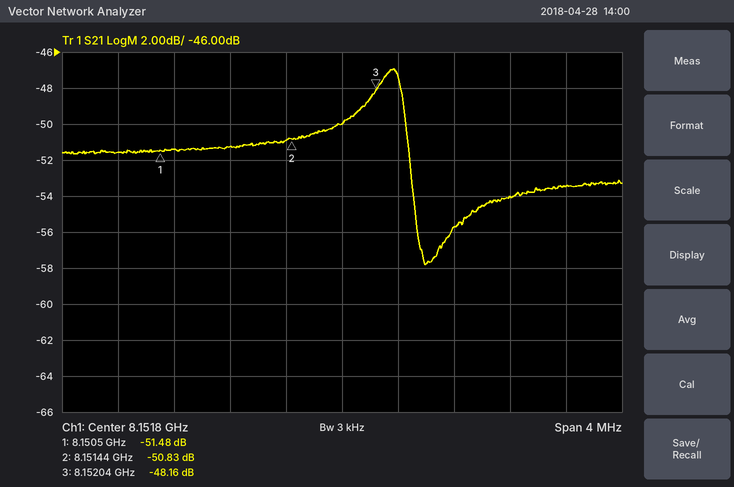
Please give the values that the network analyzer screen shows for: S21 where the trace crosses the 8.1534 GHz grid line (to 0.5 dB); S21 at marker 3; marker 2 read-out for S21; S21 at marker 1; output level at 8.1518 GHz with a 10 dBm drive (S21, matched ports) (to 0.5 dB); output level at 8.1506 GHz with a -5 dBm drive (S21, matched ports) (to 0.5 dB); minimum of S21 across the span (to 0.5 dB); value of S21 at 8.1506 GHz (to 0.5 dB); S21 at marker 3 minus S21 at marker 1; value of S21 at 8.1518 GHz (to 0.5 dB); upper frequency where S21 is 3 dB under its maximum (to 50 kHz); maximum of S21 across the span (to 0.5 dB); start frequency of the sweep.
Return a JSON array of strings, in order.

["-53.5 dB", "-48.16 dB", "-50.83 dB", "-51.48 dB", "-40.0 dBm", "-56.5 dBm", "-58.0 dB", "-51.5 dB", "3.32 dB", "-50.0 dB", "8.15225 GHz", "-47.0 dB", "8.1498 GHz"]
